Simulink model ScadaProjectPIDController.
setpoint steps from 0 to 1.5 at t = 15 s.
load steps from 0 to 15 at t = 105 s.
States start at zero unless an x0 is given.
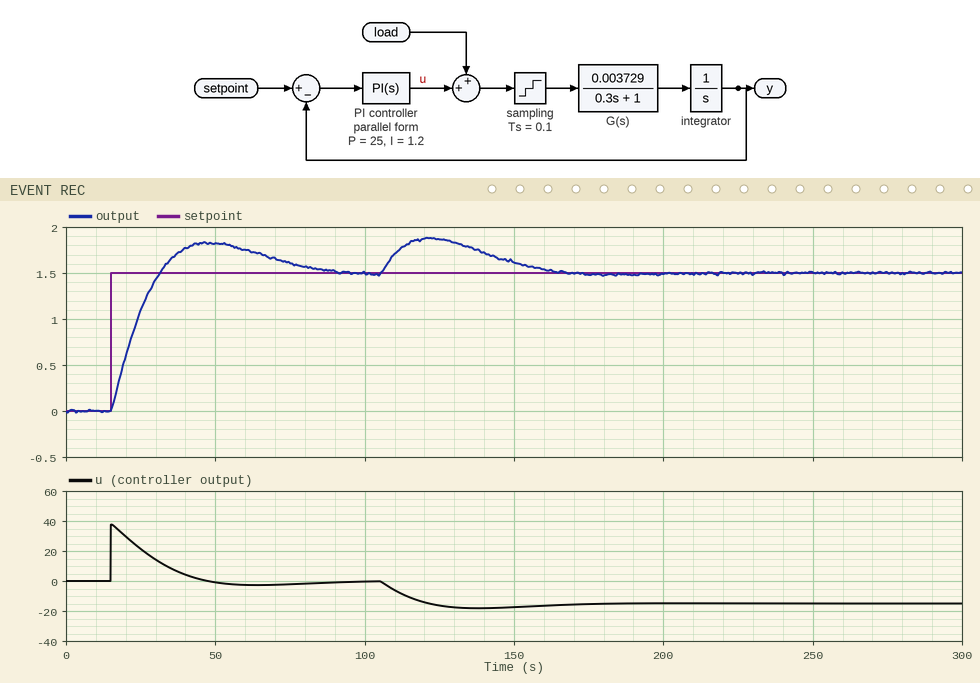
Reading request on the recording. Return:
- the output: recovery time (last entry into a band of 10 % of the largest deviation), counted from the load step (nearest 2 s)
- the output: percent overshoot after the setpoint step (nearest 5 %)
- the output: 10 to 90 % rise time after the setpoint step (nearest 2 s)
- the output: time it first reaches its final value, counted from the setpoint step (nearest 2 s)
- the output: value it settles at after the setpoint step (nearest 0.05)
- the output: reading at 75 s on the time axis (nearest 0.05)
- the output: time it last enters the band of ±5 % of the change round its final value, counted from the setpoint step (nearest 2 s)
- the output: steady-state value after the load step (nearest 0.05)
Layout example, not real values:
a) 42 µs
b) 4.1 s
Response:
a) 56 s
b) 20 %
c) 12 s
d) 16 s
e) 1.50
f) 1.60
g) 64 s
h) 1.50
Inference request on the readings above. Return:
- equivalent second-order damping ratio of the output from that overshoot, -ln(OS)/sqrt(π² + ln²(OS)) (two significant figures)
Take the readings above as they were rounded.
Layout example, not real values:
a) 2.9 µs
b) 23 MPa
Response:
a) 0.46
